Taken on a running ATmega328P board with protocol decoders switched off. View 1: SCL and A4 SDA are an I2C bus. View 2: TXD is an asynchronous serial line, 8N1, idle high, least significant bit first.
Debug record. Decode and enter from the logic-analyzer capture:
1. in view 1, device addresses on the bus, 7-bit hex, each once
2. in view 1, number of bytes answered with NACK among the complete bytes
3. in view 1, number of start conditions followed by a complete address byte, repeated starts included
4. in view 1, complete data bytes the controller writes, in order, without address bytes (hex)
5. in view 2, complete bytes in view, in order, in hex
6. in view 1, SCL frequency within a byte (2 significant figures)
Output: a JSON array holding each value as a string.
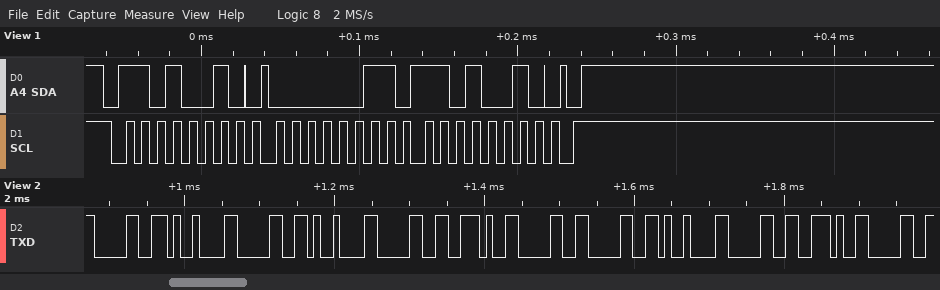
["0x69", "0", "1", "03 D2", "0x30 0x09 0x30 0x09 0x30 0x2E 0x30 0x30 0x09 0x30 0x2E 0x30", "100 kHz"]
